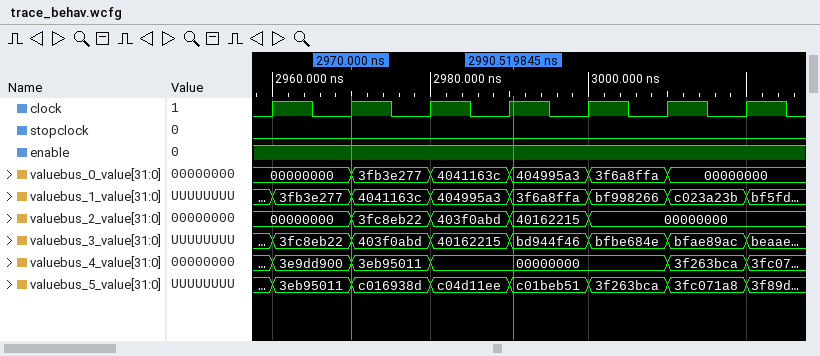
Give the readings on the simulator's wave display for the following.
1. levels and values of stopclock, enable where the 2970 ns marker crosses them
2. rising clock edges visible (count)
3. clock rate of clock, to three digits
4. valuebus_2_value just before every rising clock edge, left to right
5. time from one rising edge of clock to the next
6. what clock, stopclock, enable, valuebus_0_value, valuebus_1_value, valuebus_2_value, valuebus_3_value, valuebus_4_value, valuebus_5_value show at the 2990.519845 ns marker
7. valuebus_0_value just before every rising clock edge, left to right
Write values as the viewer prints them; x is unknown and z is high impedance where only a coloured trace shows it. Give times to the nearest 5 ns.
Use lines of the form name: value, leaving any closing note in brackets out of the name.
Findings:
levels and values of stopclock, enable where the 2970 ns marker crosses them: stopclock=0, enable=1
rising clock edges visible: 7
clock rate of clock, to three digits: 100 MHz
valuebus_2_value just before every rising clock edge, left to right: 00000000, 00000000, 3fc8eb22, 403f0abd, 40162215, 00000000, 00000000
time from one rising edge of clock to the next: 10 ns
what clock, stopclock, enable, valuebus_0_value, valuebus_1_value, valuebus_2_value, valuebus_3_value, valuebus_4_value, valuebus_5_value show at the 2990.519845 ns marker: clock=1, stopclock=0, enable=1, valuebus_0_value=404995a3, valuebus_1_value=3f6a8ffa, valuebus_2_value=40162215, valuebus_3_value=bd944f46, valuebus_4_value=00000000, valuebus_5_value=c01beb51
valuebus_0_value just before every rising clock edge, left to right: 00000000, 00000000, 3fb3e277, 4041163c, 404995a3, 3f6a8ffa, 00000000
